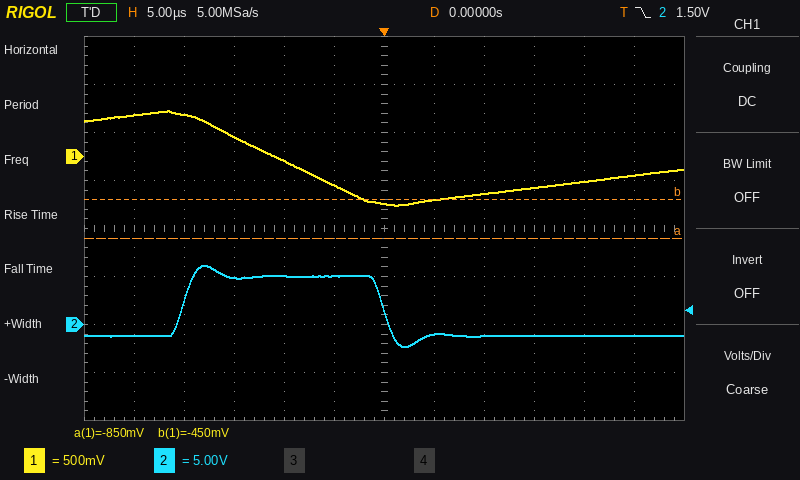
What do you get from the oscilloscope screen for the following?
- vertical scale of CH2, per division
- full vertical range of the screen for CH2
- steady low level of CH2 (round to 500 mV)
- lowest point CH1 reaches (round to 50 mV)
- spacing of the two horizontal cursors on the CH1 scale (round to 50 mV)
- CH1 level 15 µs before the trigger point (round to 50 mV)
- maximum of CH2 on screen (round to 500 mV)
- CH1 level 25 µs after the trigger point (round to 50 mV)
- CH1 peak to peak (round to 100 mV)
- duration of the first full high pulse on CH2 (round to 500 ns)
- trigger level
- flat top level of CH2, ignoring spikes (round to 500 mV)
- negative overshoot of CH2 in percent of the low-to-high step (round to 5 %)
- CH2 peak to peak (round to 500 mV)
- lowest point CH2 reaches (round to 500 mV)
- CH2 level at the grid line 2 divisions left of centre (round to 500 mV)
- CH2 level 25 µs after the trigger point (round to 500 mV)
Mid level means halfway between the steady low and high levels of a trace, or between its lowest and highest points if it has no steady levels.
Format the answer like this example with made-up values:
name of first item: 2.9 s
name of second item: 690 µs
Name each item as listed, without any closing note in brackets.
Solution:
vertical scale of CH2, per division: 5 V
full vertical range of the screen for CH2: 40 V
steady low level of CH2: -1.0 V
lowest point CH1 reaches: -500 mV
spacing of the two horizontal cursors on the CH1 scale: 400 mV
CH1 level 15 µs before the trigger point: 200 mV
maximum of CH2 on screen: 6.0 V
CH1 level 25 µs after the trigger point: -200 mV
CH1 peak to peak: 1.00 V
duration of the first full high pulse on CH2: 20.0 µs
trigger level: 1.50 V
flat top level of CH2, ignoring spikes: 5.0 V
negative overshoot of CH2 in percent of the low-to-high step: 20 %
CH2 peak to peak: 8.5 V
lowest point CH2 reaches: -2.5 V
CH2 level at the grid line 2 divisions left of centre: 5.0 V
CH2 level 25 µs after the trigger point: -1.0 V
